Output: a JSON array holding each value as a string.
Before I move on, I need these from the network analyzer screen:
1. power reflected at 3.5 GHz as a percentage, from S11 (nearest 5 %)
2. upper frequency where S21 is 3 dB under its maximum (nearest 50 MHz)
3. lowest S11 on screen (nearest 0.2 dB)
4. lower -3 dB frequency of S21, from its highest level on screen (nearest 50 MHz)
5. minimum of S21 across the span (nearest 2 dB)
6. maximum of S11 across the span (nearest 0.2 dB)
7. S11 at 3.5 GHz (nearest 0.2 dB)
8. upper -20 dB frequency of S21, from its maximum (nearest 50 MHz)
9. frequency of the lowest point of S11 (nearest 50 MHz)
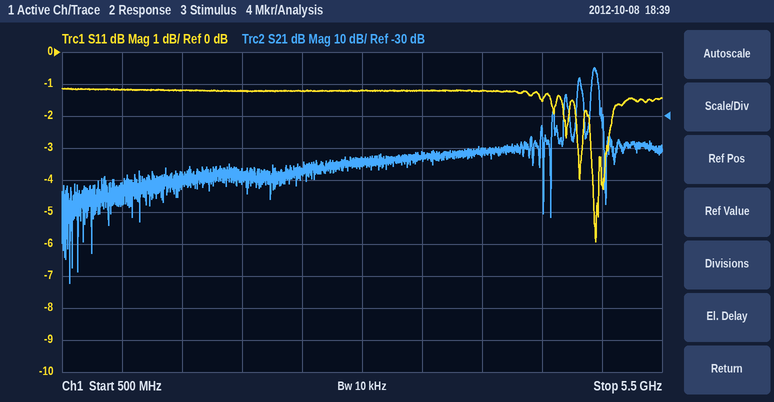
["75 %", "4.95 GHz", "-6.0 dB", "4.90 GHz", "-82 dB", "-1.2 dB", "-1.2 dB", "5.00 GHz", "4.95 GHz"]
